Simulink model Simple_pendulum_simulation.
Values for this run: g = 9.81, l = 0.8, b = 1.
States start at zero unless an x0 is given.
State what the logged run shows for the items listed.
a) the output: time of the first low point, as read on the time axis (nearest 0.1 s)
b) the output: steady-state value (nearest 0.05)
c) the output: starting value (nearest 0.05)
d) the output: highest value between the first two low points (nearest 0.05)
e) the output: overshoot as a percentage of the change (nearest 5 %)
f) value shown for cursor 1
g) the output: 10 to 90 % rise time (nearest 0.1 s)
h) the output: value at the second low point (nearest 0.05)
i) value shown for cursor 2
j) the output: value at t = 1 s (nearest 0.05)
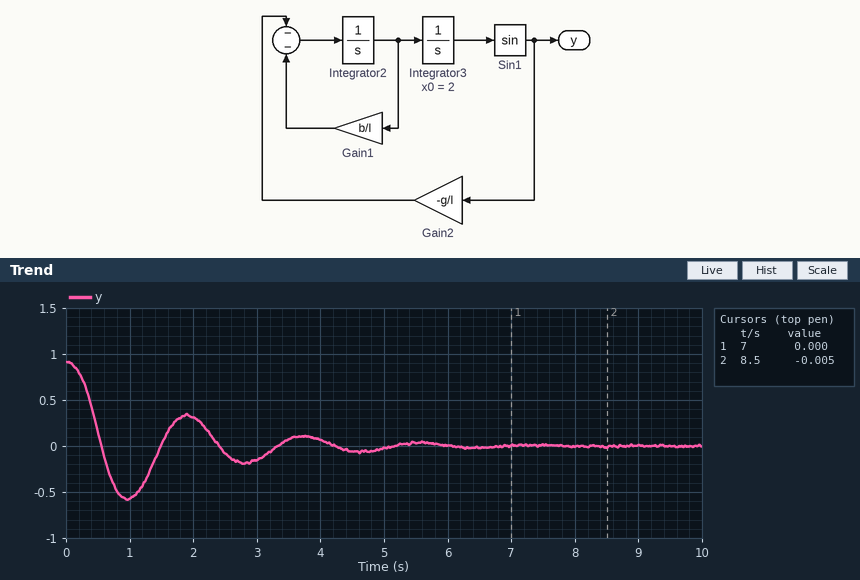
1.0 s
0.00
0.90
0.35
65 %
0.000
0.3 s
-0.20
-0.005
-0.55
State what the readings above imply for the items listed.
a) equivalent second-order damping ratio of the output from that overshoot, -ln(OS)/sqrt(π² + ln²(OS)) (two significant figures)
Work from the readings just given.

0.14
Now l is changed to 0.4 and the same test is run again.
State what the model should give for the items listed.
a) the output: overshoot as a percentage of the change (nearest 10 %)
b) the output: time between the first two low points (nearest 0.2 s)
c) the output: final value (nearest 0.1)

50 %
1.4 s
0.0
